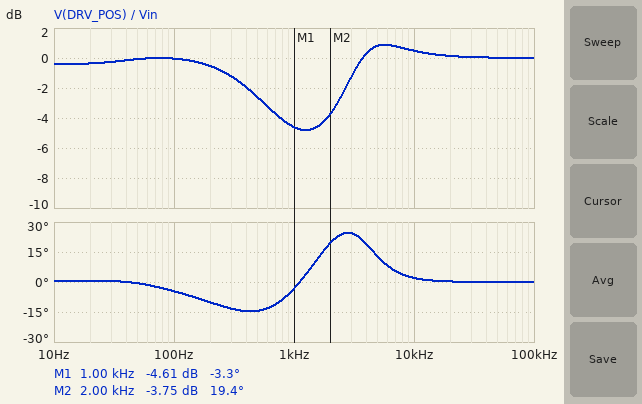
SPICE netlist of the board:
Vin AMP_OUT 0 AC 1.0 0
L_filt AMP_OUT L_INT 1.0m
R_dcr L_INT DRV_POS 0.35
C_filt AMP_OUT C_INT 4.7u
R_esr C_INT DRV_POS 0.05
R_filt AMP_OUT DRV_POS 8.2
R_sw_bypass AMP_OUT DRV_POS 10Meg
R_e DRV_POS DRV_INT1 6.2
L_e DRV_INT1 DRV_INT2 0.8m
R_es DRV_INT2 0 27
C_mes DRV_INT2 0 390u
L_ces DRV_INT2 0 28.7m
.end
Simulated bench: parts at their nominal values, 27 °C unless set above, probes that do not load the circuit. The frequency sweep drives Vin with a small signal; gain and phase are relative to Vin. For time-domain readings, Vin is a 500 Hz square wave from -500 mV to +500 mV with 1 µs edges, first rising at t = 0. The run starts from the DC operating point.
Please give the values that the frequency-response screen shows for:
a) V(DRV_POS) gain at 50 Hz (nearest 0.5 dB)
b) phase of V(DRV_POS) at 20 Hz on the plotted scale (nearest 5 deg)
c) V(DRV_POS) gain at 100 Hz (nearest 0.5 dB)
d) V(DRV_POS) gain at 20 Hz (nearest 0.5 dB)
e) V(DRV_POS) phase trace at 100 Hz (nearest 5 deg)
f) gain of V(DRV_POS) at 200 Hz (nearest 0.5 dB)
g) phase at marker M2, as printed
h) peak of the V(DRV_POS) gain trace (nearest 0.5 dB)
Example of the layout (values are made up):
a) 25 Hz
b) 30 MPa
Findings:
a) 0 dB
b) 0 deg
c) 0 dB
d) -0.5 dB
e) -5 deg
f) -0.5 dB
g) 19.4 deg
h) 1.0 dB
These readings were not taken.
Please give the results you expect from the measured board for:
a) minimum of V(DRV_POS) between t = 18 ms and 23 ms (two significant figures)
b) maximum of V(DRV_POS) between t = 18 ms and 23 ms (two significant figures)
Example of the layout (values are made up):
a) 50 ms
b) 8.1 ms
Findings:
a) -530 mV
b) 530 mV
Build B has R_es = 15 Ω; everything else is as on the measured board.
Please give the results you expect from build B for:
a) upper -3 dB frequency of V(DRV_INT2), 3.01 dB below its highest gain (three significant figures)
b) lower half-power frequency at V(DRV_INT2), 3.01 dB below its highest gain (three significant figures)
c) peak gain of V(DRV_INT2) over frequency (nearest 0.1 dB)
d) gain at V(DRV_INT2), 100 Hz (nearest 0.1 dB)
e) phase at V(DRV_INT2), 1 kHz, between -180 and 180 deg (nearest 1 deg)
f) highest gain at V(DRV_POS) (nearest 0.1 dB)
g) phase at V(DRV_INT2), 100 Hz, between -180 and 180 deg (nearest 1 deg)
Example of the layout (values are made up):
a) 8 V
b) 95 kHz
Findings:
a) 118 Hz
b) 20.9 Hz
c) -3.1 dB
d) -5.1 dB
e) -128 deg
f) 0.9 dB
g) -47 deg
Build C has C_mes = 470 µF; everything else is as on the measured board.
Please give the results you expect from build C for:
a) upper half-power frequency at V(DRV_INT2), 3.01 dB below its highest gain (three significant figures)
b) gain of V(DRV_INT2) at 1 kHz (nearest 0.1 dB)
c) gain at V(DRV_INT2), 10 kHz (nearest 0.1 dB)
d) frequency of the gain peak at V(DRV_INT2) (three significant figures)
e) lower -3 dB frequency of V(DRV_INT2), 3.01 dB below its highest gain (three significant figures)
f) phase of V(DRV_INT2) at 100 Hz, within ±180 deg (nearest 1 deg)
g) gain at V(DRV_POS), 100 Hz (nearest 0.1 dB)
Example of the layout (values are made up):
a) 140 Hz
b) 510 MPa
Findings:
a) 91.5 Hz
b) -31.8 dB
c) -63.0 dB
d) 45.4 Hz
e) 22.2 Hz
f) -59 deg
g) -0.1 dB
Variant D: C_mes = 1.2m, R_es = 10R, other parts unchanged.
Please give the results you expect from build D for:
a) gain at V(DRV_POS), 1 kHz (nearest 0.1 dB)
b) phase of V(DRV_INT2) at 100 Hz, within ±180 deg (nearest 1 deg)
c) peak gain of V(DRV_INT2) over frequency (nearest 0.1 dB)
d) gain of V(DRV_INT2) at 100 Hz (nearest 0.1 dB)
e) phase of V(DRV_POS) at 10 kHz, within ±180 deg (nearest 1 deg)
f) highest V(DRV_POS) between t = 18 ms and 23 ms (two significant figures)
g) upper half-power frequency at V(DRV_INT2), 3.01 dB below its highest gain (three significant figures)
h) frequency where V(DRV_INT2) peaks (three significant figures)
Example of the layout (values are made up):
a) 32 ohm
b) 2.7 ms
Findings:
a) -4.5 dB
b) -79 deg
c) -4.4 dB
d) -13.6 dB
e) 2 deg
f) 540 mV
g) 49.8 Hz
h) 27.6 Hz
